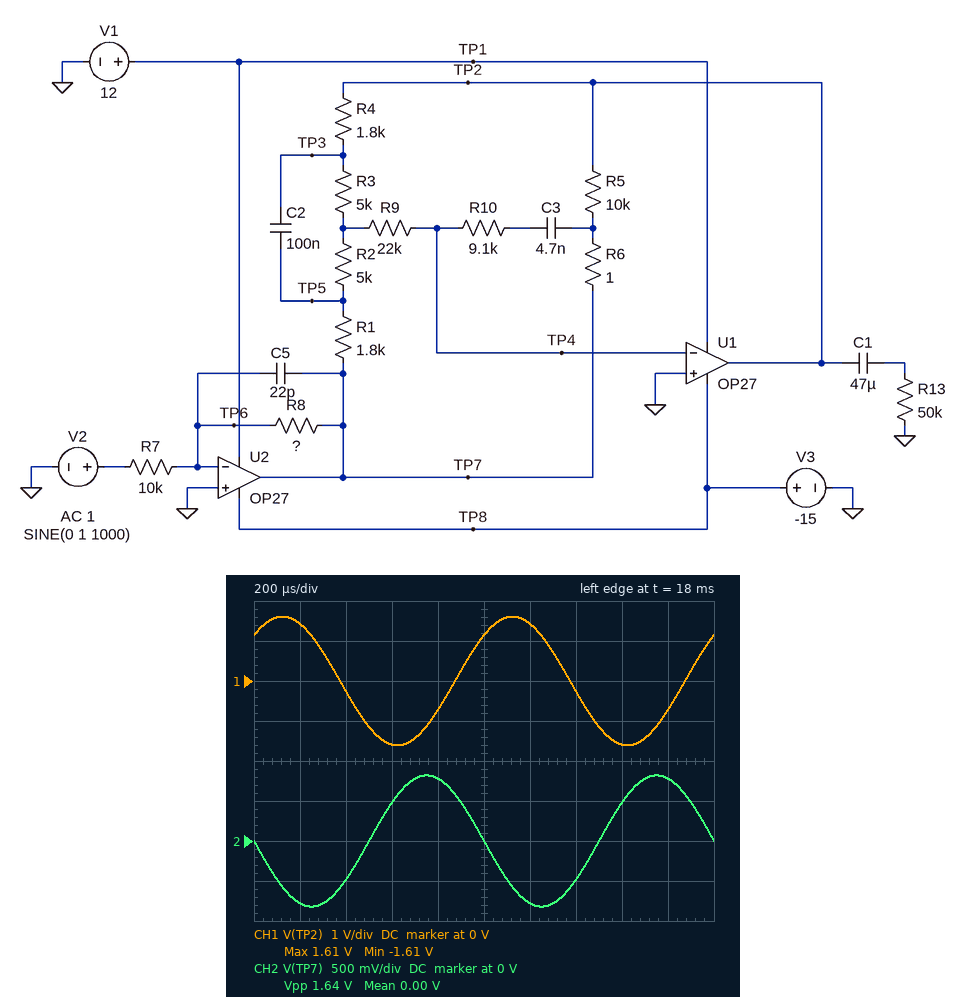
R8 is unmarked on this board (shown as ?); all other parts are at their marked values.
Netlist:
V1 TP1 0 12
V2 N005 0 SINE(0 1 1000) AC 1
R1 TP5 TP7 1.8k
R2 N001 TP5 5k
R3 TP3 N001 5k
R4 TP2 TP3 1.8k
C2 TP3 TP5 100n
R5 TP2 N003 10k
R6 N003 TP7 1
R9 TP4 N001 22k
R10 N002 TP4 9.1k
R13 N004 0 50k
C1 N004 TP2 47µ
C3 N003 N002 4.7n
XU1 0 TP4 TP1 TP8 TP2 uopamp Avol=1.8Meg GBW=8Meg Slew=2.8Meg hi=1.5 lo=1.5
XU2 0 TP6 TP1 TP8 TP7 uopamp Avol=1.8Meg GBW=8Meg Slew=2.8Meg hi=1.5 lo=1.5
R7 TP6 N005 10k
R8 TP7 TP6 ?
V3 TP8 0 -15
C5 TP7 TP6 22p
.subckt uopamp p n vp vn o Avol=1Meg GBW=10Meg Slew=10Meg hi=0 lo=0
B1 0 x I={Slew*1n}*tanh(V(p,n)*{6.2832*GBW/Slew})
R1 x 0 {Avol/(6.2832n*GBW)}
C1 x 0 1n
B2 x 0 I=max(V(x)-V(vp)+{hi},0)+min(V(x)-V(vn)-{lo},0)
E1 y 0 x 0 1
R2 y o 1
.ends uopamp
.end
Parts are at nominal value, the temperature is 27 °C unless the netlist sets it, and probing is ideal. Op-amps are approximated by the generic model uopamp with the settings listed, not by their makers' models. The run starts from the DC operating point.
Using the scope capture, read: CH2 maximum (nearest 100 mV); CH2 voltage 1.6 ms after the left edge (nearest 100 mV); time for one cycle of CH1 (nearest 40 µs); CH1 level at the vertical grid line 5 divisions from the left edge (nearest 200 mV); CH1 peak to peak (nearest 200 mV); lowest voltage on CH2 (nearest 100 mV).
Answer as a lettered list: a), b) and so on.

a) 800 mV
b) 500 mV
c) 1.00 ms
d) 1.2 V
e) 3.2 V
f) -800 mV
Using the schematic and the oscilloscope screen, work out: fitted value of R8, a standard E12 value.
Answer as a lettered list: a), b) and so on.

a) 8.2 kΩ
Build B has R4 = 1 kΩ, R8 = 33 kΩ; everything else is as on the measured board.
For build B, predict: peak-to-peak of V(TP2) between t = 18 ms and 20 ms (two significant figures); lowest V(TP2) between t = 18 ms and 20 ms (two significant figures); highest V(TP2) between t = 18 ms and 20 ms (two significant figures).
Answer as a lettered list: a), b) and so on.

a) 9.4 V
b) -4.7 V
c) 4.7 V
